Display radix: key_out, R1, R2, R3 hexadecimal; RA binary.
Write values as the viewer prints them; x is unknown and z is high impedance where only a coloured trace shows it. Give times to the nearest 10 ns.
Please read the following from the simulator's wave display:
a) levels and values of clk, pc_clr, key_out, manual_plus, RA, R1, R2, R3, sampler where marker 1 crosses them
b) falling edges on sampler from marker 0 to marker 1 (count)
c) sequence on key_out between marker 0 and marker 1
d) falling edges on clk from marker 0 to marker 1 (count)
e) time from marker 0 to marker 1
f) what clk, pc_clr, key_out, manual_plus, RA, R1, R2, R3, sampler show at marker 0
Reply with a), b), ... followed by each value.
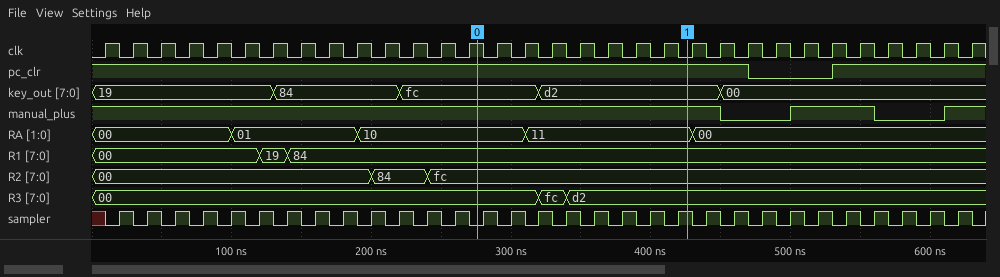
a) clk=0, pc_clr=1, key_out=d2, manual_plus=1, RA=11, R1=84, R2=fc, R3=d2, sampler=1
b) 7
c) fc, d2
d) 8
e) 150 ns
f) clk=1, pc_clr=1, key_out=fc, manual_plus=1, RA=10, R1=84, R2=fc, R3=00, sampler=0
